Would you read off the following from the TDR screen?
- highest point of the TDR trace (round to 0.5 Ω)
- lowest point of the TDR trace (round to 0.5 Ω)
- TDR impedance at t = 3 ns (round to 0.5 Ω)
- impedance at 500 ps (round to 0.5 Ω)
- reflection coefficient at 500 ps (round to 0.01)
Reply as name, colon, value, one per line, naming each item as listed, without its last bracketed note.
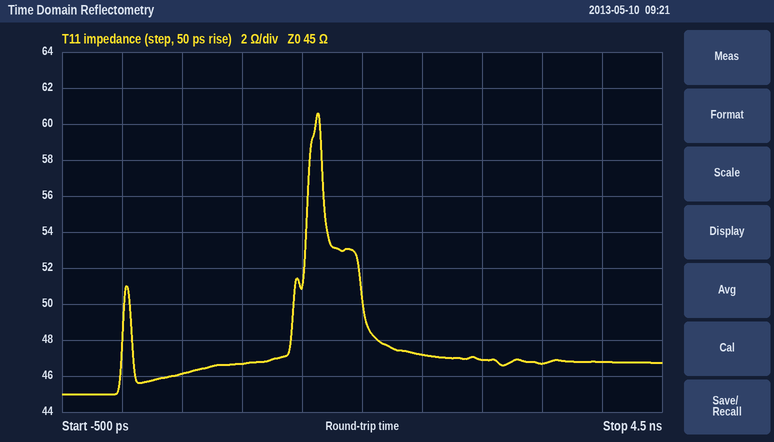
highest point of the TDR trace: 60.5 Ω
lowest point of the TDR trace: 45.0 Ω
TDR impedance at t = 3 ns: 47.0 Ω
impedance at 500 ps: 46.0 Ω
reflection coefficient at 500 ps: +0.01
